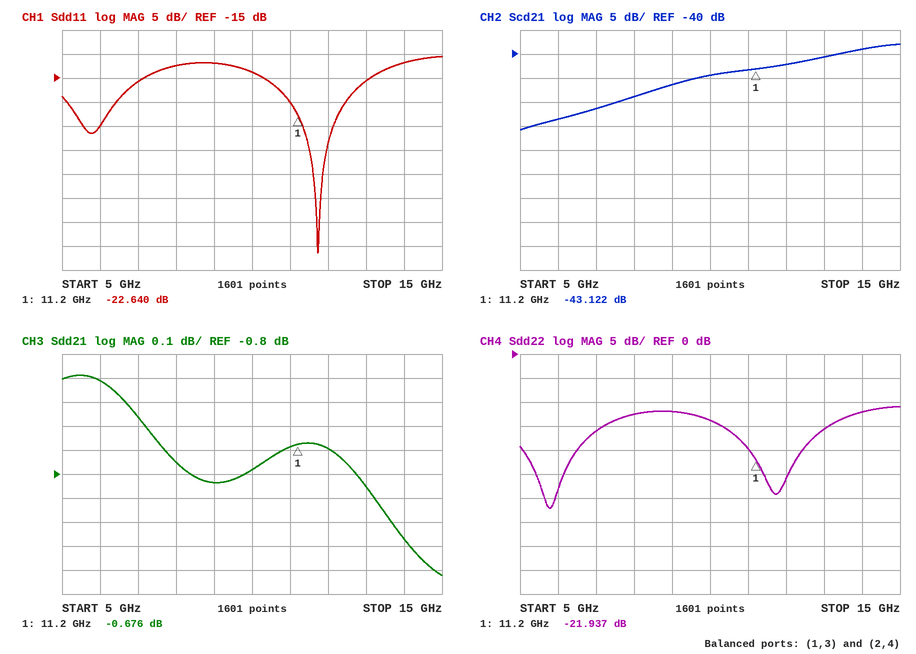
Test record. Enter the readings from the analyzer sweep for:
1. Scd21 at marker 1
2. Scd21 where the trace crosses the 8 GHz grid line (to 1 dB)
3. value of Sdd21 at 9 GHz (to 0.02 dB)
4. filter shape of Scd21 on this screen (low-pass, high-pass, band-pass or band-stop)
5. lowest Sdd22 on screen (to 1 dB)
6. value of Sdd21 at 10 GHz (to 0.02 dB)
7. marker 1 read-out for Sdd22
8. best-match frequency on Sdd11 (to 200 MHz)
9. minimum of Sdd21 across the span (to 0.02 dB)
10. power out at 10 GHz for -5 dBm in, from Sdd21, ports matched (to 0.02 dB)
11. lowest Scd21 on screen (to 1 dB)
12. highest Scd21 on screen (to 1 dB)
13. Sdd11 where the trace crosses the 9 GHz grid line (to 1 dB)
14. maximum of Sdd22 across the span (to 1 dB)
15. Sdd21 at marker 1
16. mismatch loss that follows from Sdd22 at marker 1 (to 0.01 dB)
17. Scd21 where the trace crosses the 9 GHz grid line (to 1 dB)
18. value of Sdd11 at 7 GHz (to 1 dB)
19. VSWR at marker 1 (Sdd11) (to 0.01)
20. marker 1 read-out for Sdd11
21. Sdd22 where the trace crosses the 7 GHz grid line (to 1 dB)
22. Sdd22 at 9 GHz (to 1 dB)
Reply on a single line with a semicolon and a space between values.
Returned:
-43.122 dB; -49 dB; -0.84 dB; high-pass; -32 dB; -0.78 dB; -21.937 dB; 11.8 GHz; -1.22 dB; -5.78 dBm; -56 dB; -38 dB; -12 dB; -11 dB; -0.676 dB; 0.03 dB; -46 dB; -16 dB; 1.16; -22.640 dB; -16 dB; -12 dB
